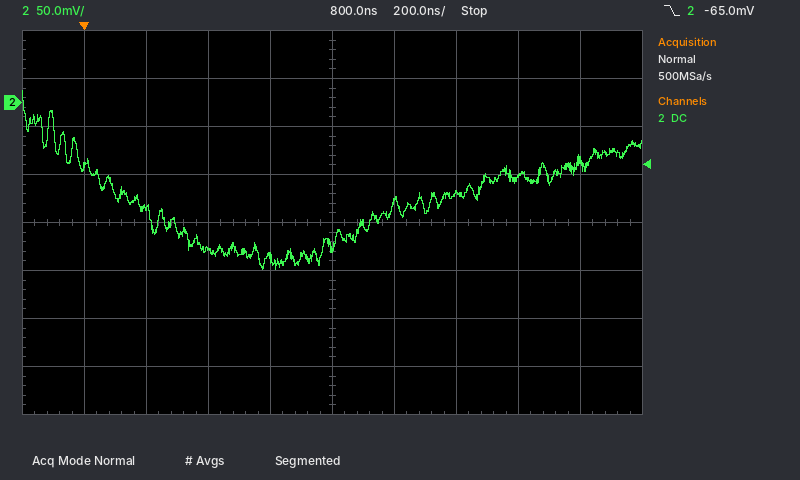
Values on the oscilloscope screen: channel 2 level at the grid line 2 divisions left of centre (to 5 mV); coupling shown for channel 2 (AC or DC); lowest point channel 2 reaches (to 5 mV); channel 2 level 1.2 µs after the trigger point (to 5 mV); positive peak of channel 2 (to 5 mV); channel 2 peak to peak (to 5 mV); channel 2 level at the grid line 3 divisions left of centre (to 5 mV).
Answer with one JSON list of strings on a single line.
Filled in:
["-155 mV", "DC", "-175 mV", "-95 mV", "10 mV", "185 mV", "-110 mV"]
